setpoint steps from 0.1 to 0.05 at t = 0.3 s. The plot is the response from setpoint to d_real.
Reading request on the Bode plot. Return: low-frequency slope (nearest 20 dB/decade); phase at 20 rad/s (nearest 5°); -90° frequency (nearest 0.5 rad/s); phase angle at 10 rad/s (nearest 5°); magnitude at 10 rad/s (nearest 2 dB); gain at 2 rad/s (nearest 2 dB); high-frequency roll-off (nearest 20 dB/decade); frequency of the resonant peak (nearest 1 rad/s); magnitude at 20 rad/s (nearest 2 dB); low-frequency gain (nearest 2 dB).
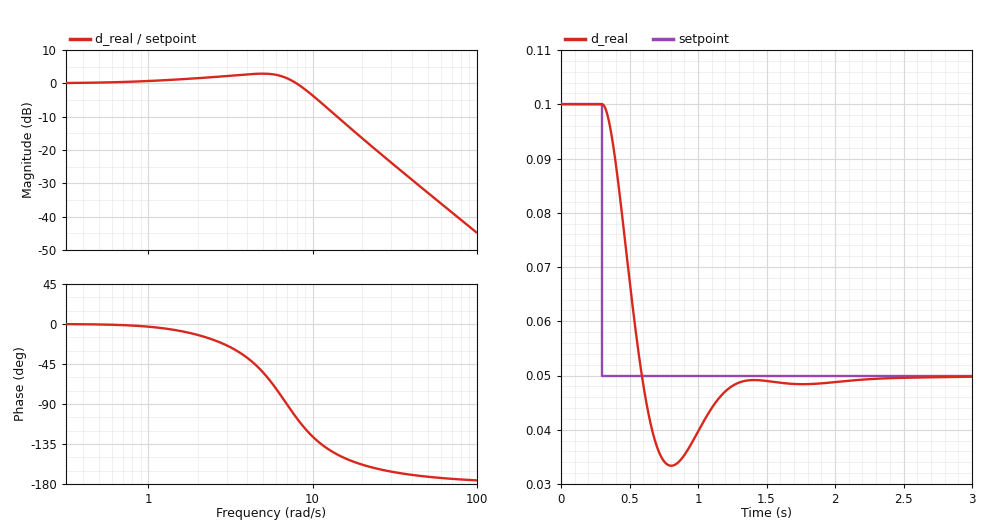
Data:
0 dB/decade
-160°
7.0 rad/s
-125°
-4 dB
2 dB
-40 dB/decade
5 rad/s
-16 dB
0 dB
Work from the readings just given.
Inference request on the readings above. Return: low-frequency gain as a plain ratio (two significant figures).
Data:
1.0
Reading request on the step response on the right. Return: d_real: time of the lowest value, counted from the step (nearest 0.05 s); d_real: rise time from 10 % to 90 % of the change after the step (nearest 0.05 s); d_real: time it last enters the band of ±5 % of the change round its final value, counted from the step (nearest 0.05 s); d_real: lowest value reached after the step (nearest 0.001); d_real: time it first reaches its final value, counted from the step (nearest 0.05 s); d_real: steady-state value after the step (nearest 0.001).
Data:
0.50 s
0.20 s
0.90 s
0.033
0.30 s
0.050
